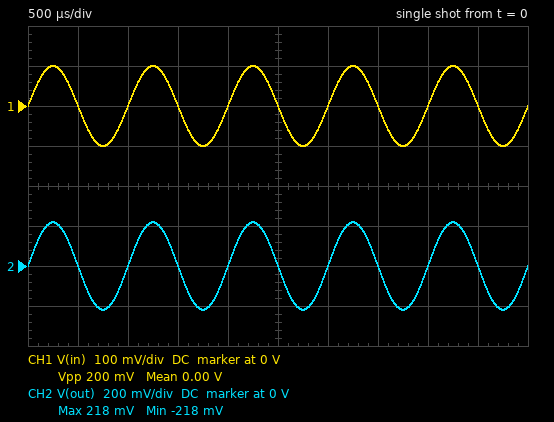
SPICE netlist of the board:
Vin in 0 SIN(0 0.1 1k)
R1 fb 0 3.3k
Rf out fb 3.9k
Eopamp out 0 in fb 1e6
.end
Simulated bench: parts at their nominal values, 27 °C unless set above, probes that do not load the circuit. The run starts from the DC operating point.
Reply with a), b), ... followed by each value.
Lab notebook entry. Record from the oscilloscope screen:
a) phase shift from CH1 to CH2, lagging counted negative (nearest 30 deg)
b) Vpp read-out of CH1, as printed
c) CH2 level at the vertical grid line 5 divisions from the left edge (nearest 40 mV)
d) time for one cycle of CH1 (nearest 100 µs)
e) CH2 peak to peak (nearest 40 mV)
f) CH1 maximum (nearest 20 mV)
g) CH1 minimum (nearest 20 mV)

a) 0 deg
b) 200 mV
c) 0 V
d) 1.0 ms
e) 440 mV
f) 100 mV
g) -100 mV
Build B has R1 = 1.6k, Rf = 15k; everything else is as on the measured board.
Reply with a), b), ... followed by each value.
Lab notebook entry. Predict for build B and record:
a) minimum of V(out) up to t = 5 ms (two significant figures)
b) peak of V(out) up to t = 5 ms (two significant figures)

a) -1.0 V
b) 1.0 V
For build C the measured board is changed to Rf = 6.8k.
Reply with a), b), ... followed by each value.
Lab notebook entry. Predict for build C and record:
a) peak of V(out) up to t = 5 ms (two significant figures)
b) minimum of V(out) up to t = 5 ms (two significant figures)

a) 310 mV
b) -310 mV
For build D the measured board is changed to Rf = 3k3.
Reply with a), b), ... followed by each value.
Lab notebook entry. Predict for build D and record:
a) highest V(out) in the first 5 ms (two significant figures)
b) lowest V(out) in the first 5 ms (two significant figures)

a) 200 mV
b) -200 mV
